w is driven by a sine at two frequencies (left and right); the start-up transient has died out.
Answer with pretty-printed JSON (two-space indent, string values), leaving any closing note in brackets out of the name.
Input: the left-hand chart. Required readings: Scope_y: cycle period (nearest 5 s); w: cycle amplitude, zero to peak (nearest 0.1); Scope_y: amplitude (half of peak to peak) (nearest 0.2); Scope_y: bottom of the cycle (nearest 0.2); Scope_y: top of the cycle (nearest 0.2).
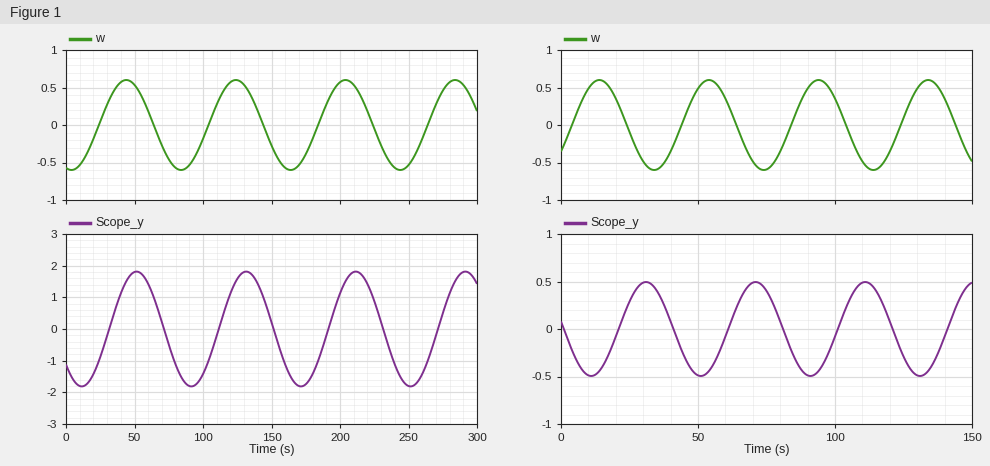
{
  "Scope_y: cycle period": "80 s",
  "w: cycle amplitude, zero to peak": "0.6",
  "Scope_y: amplitude (half of peak to peak)": "1.8",
  "Scope_y: bottom of the cycle": "-1.8",
  "Scope_y: top of the cycle": "1.8"
}
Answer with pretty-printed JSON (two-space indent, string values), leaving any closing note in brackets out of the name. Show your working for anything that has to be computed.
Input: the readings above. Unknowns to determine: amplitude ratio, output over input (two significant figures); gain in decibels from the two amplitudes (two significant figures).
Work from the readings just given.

{
  "amplitude ratio, output over input": "1.8 / 0.6 = 3.0",
  "gain in decibels from the two amplitudes": "20 log10(1.8 / 0.6) = 9.5 dB"
}
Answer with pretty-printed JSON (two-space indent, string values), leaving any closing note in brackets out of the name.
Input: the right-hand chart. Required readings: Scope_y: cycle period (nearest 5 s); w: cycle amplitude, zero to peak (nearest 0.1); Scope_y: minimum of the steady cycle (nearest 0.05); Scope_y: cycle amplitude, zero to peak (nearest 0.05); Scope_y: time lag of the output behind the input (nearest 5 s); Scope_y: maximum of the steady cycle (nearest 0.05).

{
  "Scope_y: cycle period": "40 s",
  "w: cycle amplitude, zero to peak": "0.6",
  "Scope_y: minimum of the steady cycle": "-0.50",
  "Scope_y: cycle amplitude, zero to peak": "0.50",
  "Scope_y: time lag of the output behind the input": "15 s",
  "Scope_y: maximum of the steady cycle": "0.50"
}
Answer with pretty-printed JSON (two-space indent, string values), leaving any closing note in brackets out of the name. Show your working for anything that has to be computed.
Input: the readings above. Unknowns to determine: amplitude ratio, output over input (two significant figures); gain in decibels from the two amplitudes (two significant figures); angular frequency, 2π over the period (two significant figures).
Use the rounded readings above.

{
  "amplitude ratio, output over input": "0.5 / 0.6 = 0.83",
  "gain in decibels from the two amplitudes": "20 log10(0.5 / 0.6) = -1.6 dB",
  "angular frequency, 2π over the period": "2π / 40 = 0.16 rad/s"
}
